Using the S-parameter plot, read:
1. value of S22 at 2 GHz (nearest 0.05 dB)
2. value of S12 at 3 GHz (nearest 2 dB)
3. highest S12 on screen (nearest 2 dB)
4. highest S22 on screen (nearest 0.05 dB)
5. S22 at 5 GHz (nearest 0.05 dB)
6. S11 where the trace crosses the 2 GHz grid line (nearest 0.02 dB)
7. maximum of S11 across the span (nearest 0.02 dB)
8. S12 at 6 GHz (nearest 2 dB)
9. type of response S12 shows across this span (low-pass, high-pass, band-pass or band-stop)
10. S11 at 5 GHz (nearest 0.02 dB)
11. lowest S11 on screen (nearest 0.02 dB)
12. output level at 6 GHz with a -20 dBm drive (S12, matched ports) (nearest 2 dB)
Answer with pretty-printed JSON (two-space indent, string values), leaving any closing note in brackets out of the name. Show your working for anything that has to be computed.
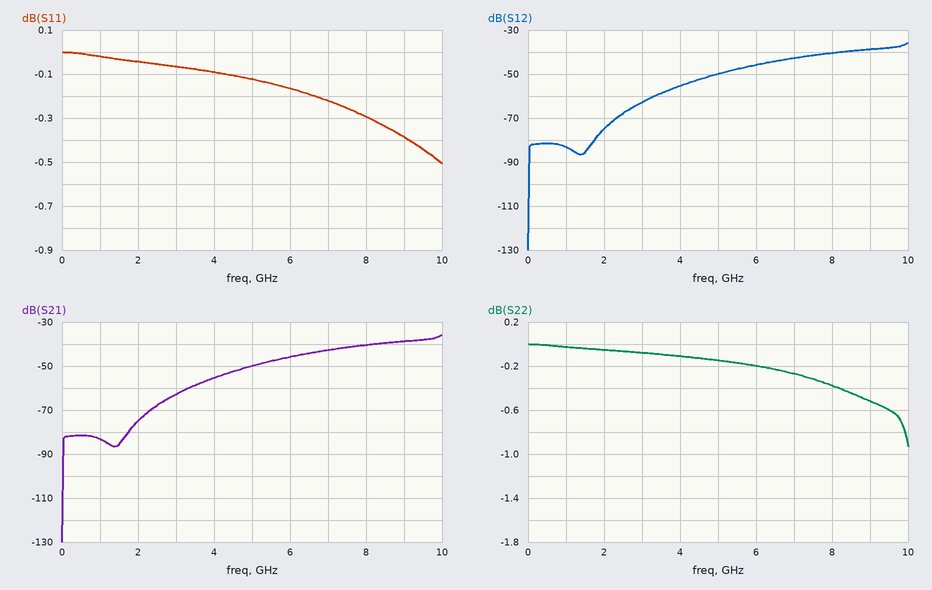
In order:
{
  "value of S22 at 2 GHz": "-0.05 dB",
  "value of S12 at 3 GHz": "-62 dB",
  "highest S12 on screen": "-36 dB",
  "highest S22 on screen": "0.00 dB",
  "S22 at 5 GHz": "-0.15 dB",
  "S11 where the trace crosses the 2 GHz grid line": "-0.04 dB",
  "maximum of S11 across the span": "0.00 dB",
  "S12 at 6 GHz": "-46 dB",
  "type of response S12 shows across this span": "high-pass",
  "S11 at 5 GHz": "-0.12 dB",
  "lowest S11 on screen": "-0.50 dB",
  "output level at 6 GHz with a -20 dBm drive (S12, matched ports)": "-20 dBm + (-46 dB) = -66 dBm"
}
